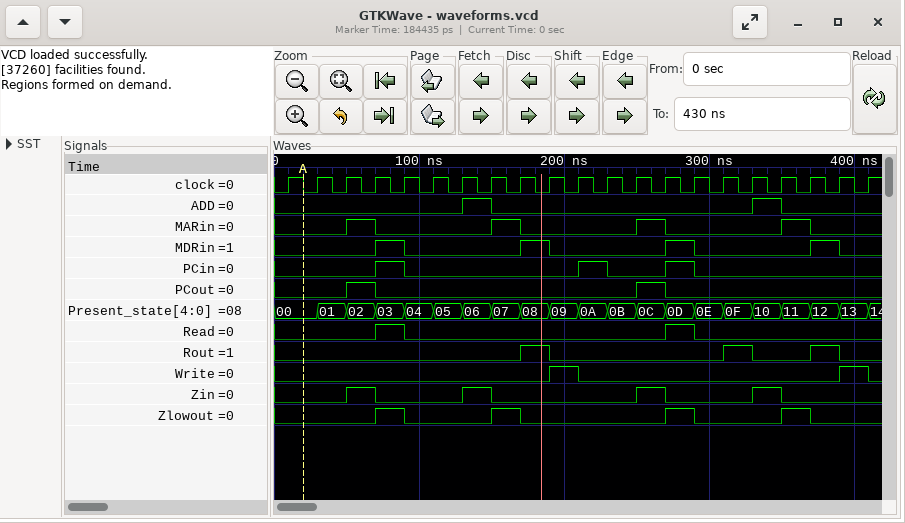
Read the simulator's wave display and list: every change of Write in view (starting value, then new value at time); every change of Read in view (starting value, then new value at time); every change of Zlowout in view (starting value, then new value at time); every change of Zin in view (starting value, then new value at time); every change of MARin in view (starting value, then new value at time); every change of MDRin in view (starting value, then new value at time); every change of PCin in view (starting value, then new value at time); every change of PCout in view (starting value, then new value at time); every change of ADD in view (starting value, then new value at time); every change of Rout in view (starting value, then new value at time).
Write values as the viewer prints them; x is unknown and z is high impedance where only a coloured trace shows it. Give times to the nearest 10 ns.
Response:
0, 1 at 190 ns, 0 at 210 ns, 1 at 390 ns, 0 at 410 ns
0, 1 at 70 ns, 0 at 90 ns, 1 at 270 ns, 0 at 290 ns
0, 1 at 70 ns, 0 at 90 ns, 1 at 150 ns, 0 at 170 ns, 1 at 270 ns, 0 at 290 ns, 1 at 350 ns, 0 at 370 ns
0, 1 at 50 ns, 0 at 70 ns, 1 at 130 ns, 0 at 150 ns, 1 at 250 ns, 0 at 270 ns, 1 at 330 ns, 0 at 350 ns
0, 1 at 50 ns, 0 at 70 ns, 1 at 150 ns, 0 at 170 ns, 1 at 250 ns, 0 at 270 ns, 1 at 350 ns, 0 at 370 ns
0, 1 at 70 ns, 0 at 90 ns, 1 at 170 ns, 0 at 190 ns, 1 at 270 ns, 0 at 290 ns, 1 at 370 ns, 0 at 390 ns
0, 1 at 70 ns, 0 at 90 ns, 1 at 210 ns, 0 at 230 ns, 1 at 270 ns, 0 at 290 ns
0, 1 at 50 ns, 0 at 70 ns, 1 at 250 ns, 0 at 270 ns
0, 1 at 130 ns, 0 at 150 ns, 1 at 330 ns, 0 at 350 ns
0, 1 at 170 ns, 0 at 190 ns, 1 at 310 ns, 0 at 330 ns, 1 at 370 ns, 0 at 390 ns
